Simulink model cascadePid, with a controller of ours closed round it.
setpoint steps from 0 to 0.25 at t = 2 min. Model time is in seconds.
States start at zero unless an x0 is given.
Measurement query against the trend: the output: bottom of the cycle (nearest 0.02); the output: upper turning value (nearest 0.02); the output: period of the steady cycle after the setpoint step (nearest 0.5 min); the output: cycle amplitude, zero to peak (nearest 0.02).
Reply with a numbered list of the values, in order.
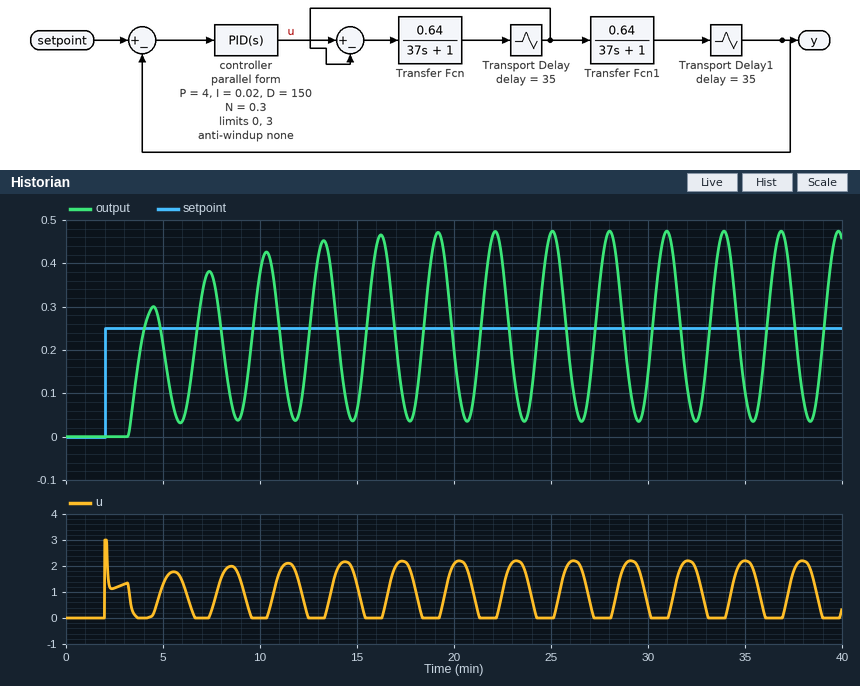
1. 0.04
2. 0.48
3. 3.0 min
4. 0.22
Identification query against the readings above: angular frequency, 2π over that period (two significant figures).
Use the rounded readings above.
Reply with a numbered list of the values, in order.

1. 2.1 rad/min
